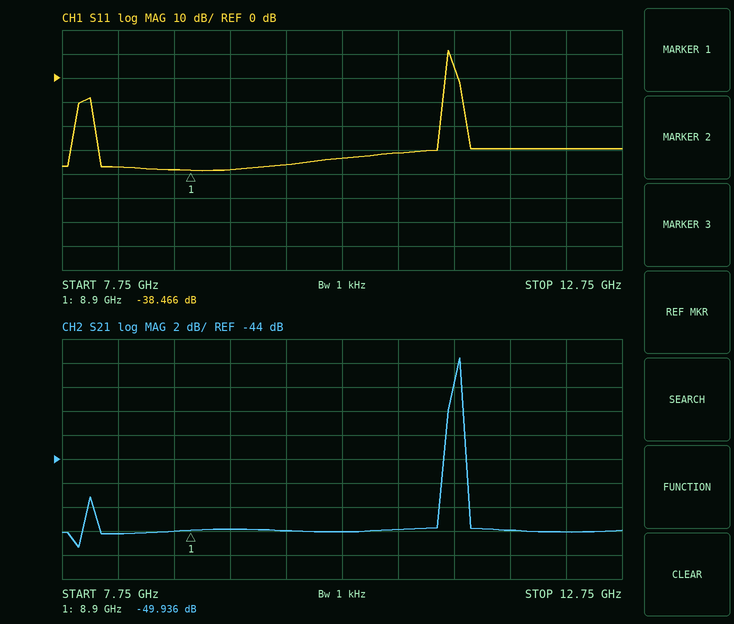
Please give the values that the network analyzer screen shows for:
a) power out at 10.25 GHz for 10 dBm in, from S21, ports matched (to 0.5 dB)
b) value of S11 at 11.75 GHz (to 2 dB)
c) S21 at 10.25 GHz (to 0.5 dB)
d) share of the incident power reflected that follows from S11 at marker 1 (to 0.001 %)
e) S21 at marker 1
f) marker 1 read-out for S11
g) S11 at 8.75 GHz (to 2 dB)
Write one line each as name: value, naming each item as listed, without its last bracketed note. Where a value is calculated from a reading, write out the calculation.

power out at 10.25 GHz for 10 dBm in, from S21, ports matched: 10 dBm + (-50.0 dB) = -40.0 dBm
value of S11 at 11.75 GHz: -30 dB
S21 at 10.25 GHz: -50.0 dB
share of the incident power reflected that follows from S11 at marker 1: 10^(-38.466/10) ≈ 0.014 %
S21 at marker 1: -49.936 dB
marker 1 read-out for S11: -38.466 dB
S11 at 8.75 GHz: -38 dB
